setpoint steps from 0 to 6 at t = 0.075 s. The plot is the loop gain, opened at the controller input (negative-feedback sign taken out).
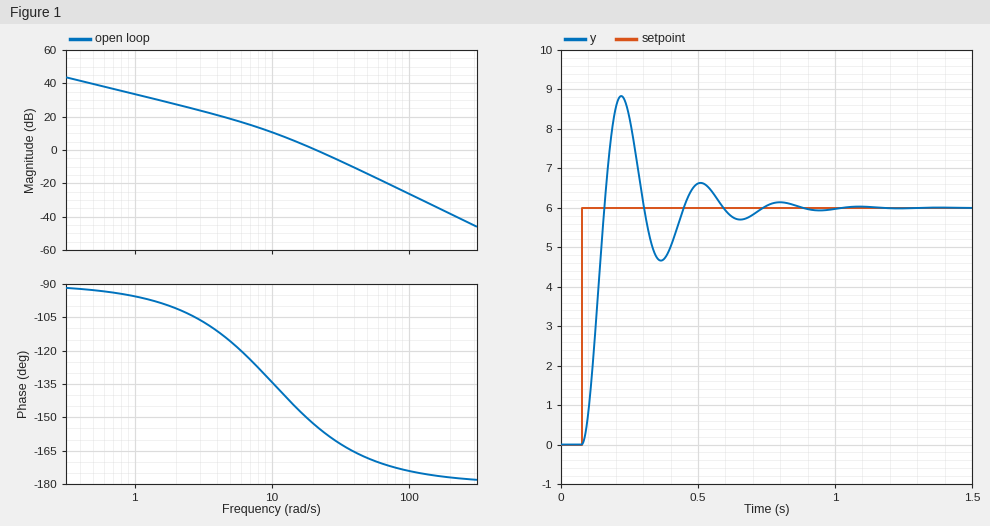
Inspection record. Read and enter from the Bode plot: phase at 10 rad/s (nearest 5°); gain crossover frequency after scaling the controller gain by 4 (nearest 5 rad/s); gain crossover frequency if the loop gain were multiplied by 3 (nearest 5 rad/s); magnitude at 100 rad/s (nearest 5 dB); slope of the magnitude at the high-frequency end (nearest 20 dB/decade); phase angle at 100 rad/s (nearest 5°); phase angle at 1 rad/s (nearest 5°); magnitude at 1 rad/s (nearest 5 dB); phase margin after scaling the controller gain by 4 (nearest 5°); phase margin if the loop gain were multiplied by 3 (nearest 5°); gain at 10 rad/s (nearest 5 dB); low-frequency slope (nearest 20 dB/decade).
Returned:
-135°
45 rad/s
40 rad/s
-25 dB
-40 dB/decade
-175°
-95°
35 dB
15°
15°
10 dB
-20 dB/decade
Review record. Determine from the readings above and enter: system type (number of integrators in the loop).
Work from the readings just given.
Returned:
1
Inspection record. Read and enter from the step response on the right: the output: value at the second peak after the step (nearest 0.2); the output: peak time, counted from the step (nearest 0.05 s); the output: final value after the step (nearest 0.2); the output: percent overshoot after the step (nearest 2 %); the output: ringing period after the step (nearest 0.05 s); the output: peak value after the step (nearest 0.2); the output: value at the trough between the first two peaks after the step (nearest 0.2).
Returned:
6.6
0.15 s
6.0
48 %
0.30 s
8.8
4.6
